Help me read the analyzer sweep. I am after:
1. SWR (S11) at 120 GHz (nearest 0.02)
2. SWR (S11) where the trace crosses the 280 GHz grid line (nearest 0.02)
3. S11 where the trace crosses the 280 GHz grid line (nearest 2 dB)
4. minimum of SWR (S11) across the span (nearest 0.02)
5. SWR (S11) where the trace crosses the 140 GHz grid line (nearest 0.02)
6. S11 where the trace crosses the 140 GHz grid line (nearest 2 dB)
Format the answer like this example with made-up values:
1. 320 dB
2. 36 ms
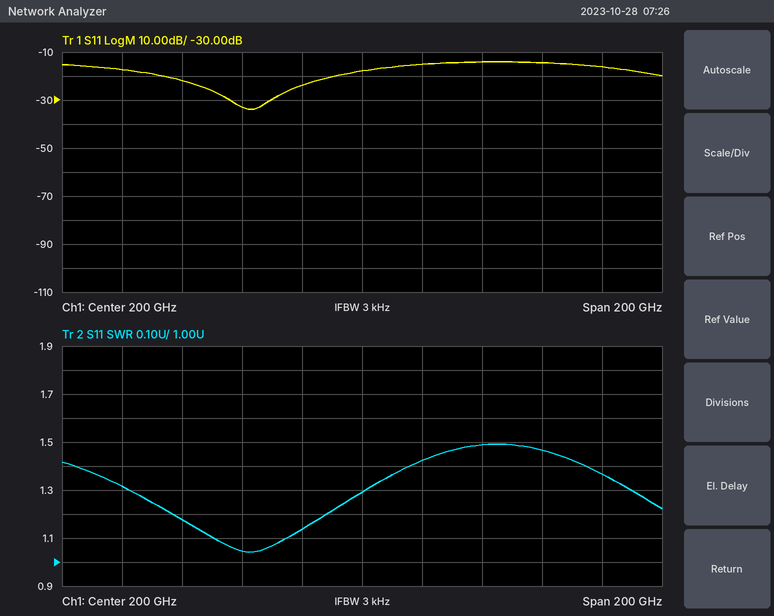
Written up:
1. 1.32
2. 1.36
3. -16 dB
4. 1.04
5. 1.18
6. -22 dB
